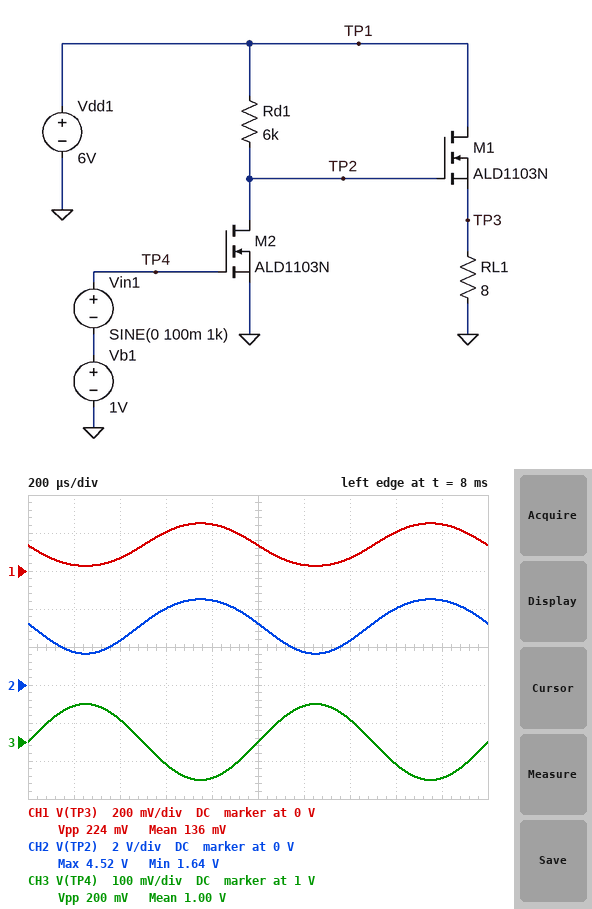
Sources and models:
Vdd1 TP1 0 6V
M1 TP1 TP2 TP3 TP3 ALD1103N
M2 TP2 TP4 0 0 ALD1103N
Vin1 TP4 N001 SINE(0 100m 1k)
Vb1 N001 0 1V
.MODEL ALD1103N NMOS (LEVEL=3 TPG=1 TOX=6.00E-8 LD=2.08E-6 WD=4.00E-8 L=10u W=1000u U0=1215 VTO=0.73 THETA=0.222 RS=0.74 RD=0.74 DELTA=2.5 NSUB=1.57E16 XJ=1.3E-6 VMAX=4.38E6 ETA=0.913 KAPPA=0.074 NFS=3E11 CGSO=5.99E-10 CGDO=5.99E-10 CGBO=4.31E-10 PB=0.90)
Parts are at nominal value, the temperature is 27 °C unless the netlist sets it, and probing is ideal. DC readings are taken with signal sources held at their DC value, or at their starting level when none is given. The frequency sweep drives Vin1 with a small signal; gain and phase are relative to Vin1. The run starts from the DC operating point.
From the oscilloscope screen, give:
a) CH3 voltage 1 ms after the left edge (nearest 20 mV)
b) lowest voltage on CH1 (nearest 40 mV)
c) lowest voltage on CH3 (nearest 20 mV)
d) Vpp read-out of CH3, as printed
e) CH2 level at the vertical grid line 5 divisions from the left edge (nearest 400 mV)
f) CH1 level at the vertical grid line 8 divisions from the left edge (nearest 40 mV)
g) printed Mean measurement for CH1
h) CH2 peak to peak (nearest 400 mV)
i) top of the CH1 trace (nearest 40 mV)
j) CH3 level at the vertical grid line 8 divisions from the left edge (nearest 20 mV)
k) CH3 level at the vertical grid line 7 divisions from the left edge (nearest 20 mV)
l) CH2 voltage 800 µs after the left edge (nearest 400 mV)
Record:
1.00 V
40 mV
900 mV
200 mV
3.2 V
200 mV
136 mV
2.8 V
240 mV
940 mV
1.06 V
4.4 V
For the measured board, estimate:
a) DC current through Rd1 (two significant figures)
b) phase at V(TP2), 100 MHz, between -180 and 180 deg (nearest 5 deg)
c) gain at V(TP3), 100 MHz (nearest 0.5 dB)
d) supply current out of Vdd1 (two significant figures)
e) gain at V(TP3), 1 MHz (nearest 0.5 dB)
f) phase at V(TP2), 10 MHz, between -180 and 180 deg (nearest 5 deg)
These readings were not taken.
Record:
460 µA
85 deg
-20.5 dB
17 mA
1.5 dB
125 deg
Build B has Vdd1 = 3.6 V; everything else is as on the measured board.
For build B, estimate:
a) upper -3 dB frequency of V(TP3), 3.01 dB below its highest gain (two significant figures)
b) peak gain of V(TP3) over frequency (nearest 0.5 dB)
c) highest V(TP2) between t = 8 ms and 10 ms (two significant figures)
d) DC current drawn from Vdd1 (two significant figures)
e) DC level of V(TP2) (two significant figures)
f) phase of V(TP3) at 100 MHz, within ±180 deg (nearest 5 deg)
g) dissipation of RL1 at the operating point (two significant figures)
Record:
7.4 MHz
-9.5 dB
2.3 V
1.0 mA
1.1 V
115 deg
3.0 µW
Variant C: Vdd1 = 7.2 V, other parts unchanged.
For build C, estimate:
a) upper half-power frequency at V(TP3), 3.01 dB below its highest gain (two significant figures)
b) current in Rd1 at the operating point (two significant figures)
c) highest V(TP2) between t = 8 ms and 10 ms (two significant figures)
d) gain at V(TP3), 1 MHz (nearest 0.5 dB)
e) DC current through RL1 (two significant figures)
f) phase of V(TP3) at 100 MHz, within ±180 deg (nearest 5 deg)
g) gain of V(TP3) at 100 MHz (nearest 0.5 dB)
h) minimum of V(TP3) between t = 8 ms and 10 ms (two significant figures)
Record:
7.8 MHz
480 µA
5.6 V
3.0 dB
29 mA
95 deg
-19.0 dB
94 mV
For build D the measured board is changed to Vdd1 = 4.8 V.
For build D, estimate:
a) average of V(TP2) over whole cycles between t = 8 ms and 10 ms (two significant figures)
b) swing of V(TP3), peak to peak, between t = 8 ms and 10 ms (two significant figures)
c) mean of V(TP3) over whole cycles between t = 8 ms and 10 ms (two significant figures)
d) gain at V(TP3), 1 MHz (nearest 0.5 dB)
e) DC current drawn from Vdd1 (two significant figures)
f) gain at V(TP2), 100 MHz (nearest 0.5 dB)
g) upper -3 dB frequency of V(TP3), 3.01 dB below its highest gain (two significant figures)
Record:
2.1 V
150 mV
64 mV
-1.0 dB
7.3 mA
0.5 dB
7.6 MHz
